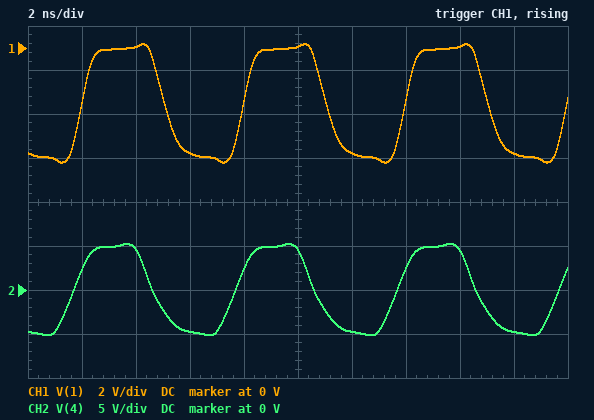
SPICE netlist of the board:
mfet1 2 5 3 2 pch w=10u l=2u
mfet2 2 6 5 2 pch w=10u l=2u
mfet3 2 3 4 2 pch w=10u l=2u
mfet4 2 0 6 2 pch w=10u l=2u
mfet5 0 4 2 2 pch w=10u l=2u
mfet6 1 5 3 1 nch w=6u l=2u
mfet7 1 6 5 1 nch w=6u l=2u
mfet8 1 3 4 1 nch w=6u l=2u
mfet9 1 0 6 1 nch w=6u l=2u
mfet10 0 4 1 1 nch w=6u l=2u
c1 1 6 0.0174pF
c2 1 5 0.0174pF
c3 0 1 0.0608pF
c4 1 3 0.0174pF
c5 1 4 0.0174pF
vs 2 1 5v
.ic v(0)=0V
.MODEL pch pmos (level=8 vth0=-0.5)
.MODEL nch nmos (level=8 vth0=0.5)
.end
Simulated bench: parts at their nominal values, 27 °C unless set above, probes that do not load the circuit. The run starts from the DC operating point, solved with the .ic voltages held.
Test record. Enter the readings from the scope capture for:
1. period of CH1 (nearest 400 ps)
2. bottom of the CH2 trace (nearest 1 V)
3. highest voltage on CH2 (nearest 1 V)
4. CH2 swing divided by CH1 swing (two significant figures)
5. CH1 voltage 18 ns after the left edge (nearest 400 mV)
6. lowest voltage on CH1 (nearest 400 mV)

6.0 ns
-5 V
5 V
1.9
-4.8 V
-5.2 V
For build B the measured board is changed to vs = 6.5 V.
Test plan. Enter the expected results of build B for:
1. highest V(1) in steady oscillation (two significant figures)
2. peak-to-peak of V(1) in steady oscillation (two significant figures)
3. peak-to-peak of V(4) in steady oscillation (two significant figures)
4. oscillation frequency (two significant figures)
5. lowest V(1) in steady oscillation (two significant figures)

180 mV
6.9 V
13 V
200 MHz
-6.7 V
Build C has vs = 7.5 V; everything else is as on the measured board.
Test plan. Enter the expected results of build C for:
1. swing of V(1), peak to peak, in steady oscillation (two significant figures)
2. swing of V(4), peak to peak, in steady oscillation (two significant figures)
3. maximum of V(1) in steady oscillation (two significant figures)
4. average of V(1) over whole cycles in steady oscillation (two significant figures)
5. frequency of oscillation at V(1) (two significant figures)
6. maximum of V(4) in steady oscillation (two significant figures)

7.9 V
15 V
190 mV
-3.6 V
220 MHz
7.8 V
